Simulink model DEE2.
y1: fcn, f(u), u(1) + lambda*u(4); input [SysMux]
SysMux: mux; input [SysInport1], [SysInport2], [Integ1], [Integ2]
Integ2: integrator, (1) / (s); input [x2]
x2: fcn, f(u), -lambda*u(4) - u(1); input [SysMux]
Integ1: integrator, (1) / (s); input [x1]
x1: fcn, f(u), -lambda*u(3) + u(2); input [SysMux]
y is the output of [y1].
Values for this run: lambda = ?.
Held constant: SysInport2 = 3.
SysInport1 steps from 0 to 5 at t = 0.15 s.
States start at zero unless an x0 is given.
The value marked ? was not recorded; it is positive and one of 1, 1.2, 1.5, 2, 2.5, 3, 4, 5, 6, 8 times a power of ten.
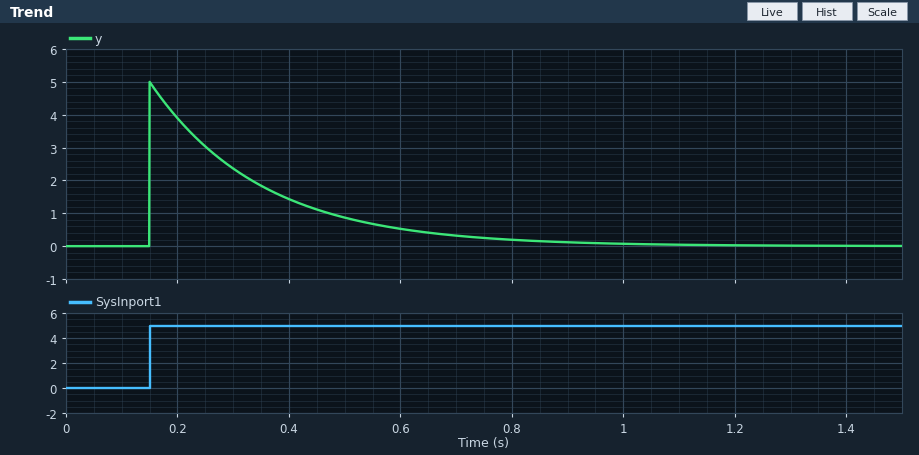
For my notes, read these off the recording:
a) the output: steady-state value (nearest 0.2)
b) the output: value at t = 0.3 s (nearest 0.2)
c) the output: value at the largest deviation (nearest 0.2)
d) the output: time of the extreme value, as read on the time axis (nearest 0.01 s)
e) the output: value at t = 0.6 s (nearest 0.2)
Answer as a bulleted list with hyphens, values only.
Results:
- 0.0
- 2.4
- 5.0
- 0.15 s
- 0.6
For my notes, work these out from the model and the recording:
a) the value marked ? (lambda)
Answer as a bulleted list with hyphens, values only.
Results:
- 5
